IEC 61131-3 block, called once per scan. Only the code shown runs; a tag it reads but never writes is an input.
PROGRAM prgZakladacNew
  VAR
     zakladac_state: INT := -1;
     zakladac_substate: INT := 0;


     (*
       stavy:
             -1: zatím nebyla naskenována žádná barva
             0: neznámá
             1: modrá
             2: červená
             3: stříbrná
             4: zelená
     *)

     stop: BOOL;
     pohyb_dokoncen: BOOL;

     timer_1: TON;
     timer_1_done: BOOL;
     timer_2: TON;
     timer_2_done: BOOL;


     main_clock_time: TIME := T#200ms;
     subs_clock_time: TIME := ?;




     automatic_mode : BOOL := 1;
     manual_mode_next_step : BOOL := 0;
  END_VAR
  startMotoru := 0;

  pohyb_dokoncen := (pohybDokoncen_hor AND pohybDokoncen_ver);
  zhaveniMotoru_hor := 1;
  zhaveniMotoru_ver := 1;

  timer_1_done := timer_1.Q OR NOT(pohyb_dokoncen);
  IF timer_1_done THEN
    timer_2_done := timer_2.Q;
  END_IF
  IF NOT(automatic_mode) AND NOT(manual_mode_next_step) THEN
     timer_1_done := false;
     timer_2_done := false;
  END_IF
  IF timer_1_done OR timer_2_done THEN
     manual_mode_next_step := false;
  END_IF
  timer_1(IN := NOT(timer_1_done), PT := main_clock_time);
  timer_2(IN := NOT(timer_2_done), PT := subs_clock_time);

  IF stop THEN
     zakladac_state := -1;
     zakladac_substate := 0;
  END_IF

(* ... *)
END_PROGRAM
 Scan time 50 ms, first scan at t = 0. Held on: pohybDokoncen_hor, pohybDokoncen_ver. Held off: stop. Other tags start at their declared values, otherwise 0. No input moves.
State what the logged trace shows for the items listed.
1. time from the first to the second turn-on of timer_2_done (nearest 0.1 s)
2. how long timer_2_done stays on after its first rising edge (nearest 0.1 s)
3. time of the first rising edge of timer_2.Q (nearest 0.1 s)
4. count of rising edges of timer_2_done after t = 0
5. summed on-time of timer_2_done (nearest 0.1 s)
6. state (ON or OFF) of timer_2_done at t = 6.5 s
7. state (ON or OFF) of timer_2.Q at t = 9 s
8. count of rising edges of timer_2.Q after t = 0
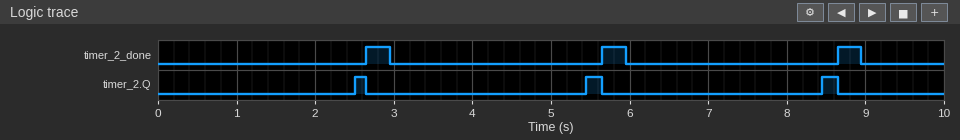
3.0 s
0.3 s
2.5 s
3
0.9 s
OFF
OFF
3
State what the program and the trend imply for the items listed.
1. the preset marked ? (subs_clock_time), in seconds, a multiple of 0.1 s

2.5 s
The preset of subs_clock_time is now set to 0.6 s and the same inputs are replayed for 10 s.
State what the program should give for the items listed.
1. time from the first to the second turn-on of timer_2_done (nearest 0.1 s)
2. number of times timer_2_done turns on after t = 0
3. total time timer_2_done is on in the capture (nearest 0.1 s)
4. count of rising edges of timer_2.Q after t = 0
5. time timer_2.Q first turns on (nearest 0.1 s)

1.2 s
8
2.4 s
8
0.6 s
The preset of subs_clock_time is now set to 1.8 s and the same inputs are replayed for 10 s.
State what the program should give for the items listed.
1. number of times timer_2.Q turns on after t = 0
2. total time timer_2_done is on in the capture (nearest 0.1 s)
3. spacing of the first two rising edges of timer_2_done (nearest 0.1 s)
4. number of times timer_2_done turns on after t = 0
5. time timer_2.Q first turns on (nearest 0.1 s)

4
1.2 s
2.4 s
4
1.8 s
